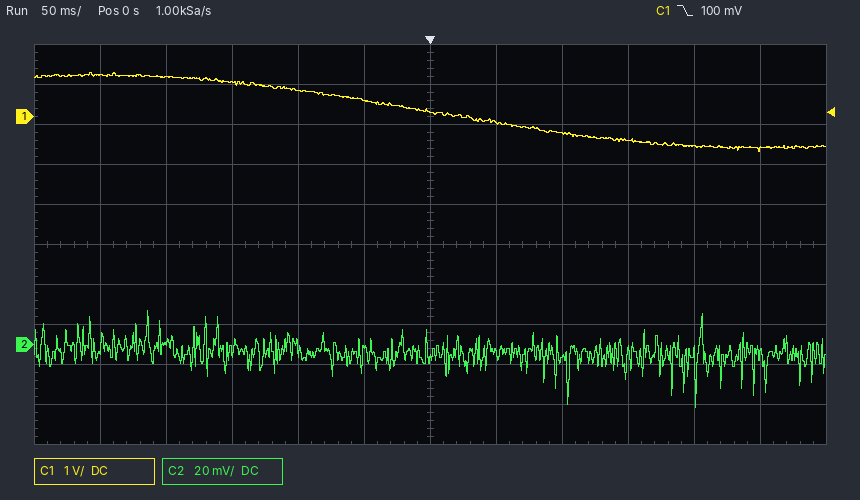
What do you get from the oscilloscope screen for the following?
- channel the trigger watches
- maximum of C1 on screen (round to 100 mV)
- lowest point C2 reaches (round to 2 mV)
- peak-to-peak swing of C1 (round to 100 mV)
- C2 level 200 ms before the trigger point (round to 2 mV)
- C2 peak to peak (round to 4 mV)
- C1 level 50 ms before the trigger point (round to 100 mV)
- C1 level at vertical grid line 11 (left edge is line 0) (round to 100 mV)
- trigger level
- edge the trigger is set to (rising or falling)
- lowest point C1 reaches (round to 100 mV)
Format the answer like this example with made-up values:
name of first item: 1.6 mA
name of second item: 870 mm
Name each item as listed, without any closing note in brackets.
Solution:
channel the trigger watches: C1
maximum of C1 on screen: 1.1 V
lowest point C2 reaches: -32 mV
peak-to-peak swing of C1: 2.0 V
C2 level 200 ms before the trigger point: 2 mV
C2 peak to peak: 48 mV
C1 level 50 ms before the trigger point: 400 mV
C1 level at vertical grid line 11 (left edge is line 0): -800 mV
trigger level: 100 mV
edge the trigger is set to: falling
lowest point C1 reaches: -900 mV
